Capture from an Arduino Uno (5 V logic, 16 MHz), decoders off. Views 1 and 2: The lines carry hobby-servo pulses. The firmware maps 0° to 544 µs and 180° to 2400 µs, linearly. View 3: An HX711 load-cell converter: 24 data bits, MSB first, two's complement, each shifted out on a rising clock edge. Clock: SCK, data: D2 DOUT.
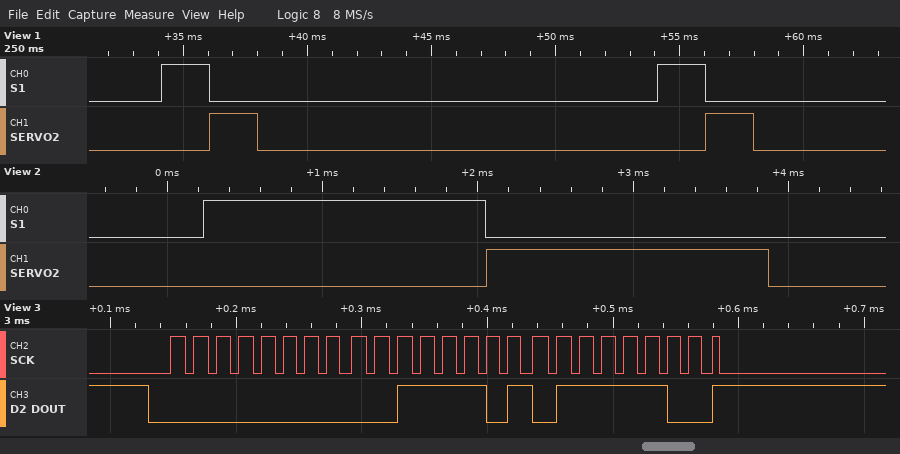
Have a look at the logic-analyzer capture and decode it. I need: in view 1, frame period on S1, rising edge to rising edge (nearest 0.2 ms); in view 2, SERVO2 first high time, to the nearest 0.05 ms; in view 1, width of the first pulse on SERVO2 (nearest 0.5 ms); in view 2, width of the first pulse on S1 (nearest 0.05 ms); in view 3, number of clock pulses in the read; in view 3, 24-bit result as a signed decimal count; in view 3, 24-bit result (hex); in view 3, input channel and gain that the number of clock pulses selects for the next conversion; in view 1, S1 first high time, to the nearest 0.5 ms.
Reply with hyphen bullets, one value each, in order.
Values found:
- 20.0 ms
- 1.80 ms
- 2.0 ms
- 1.80 ms
- 25
- 15740
- 0x003D7C
- channel A, gain 128
- 2.0 ms
